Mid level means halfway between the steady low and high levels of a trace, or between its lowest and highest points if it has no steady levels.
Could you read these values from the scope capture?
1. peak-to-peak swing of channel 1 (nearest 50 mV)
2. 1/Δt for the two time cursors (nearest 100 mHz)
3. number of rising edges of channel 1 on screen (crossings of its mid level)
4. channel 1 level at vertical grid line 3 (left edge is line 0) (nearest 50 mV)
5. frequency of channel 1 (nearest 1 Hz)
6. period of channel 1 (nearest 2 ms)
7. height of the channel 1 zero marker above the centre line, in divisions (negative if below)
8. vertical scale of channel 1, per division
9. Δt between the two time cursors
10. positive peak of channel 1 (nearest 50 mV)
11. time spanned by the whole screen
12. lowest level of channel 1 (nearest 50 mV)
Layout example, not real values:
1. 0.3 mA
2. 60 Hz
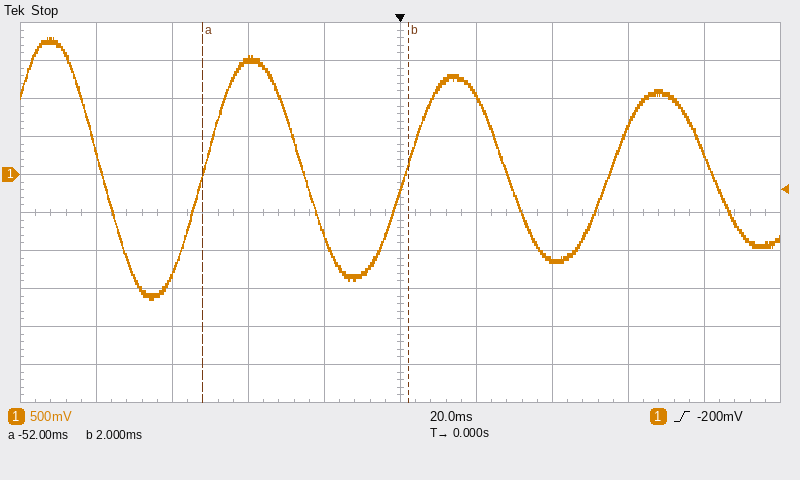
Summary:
1. 3.45 V
2. 18.5 Hz
3. 3
4. 1.50 V
5. 19 Hz
6. 54 ms
7. +1.0 div
8. 500 mV
9. 54 ms
10. 1.80 V
11. 200 ms
12. -1.65 V
